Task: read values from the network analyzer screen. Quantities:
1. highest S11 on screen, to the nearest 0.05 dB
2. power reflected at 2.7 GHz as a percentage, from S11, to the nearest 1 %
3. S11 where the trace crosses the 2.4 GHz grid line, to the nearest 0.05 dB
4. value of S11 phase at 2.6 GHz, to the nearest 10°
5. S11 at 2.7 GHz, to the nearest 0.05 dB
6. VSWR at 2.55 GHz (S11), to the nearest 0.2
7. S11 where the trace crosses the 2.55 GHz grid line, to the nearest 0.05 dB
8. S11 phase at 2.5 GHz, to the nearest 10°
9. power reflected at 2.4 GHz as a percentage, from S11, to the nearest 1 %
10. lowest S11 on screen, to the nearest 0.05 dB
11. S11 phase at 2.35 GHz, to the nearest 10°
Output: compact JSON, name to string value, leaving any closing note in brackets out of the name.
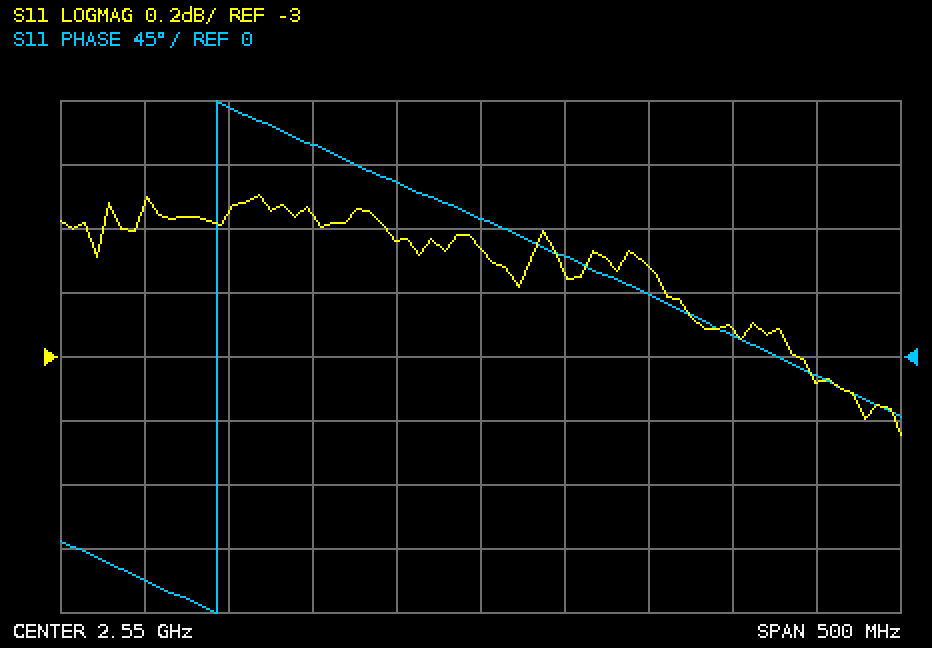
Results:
{"highest S11 on screen, to the nearest 0.05 dB": "-2.50 dB", "power reflected at 2.7 GHz as a percentage, from S11, to the nearest 1 %": "51 %", "S11 where the trace crosses the 2.4 GHz grid line, to the nearest 0.05 dB": "-2.55 dB", "value of S11 phase at 2.6 GHz, to the nearest 10°": "70°", "S11 at 2.7 GHz, to the nearest 0.05 dB": "-2.90 dB", "VSWR at 2.55 GHz (S11), to the nearest 0.2": "6.6", "S11 where the trace crosses the 2.55 GHz grid line, to the nearest 0.05 dB": "-2.65 dB", "S11 phase at 2.5 GHz, to the nearest 10°": "120°", "power reflected at 2.4 GHz as a percentage, from S11, to the nearest 1 %": "56 %", "lowest S11 on screen, to the nearest 0.05 dB": "-3.25 dB", "S11 phase at 2.35 GHz, to the nearest 10°": "-160°"}
